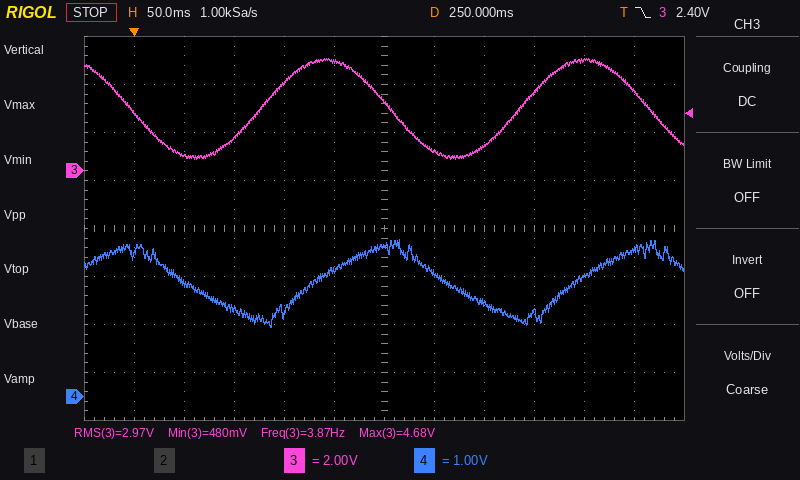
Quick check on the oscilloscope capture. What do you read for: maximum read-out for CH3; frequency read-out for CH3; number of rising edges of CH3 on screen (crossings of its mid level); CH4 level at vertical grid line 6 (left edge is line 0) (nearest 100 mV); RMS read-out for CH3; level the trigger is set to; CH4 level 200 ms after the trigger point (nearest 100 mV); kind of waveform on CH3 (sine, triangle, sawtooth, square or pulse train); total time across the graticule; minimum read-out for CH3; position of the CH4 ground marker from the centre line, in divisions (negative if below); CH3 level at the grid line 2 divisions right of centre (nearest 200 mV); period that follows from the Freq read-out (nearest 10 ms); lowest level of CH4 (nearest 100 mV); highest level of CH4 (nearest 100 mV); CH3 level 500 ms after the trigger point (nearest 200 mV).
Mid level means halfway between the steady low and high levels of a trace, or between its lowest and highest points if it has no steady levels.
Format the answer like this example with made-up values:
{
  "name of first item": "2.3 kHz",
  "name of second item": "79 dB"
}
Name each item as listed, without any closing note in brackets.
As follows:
{
  "maximum read-out for CH3": "4.68 V",
  "frequency read-out for CH3": "3.87 Hz",
  "number of rising edges of CH3 on screen": "2",
  "CH4 level at vertical grid line 6 (left edge is line 0)": "3.1 V",
  "RMS read-out for CH3": "2.97 V",
  "level the trigger is set to": "2.40 V",
  "CH4 level 200 ms after the trigger point": "2.6 V",
  "kind of waveform on CH3": "sine",
  "total time across the graticule": "600 ms",
  "minimum read-out for CH3": "480 mV",
  "position of the CH4 ground marker from the centre line, in divisions": "-3.5 div",
  "CH3 level at the grid line 2 divisions right of centre": "1.0 V",
  "period that follows from the Freq read-out": "260 ms",
  "lowest level of CH4": "1.4 V",
  "highest level of CH4": "3.3 V",
  "CH3 level 500 ms after the trigger point": "3.4 V"
}
